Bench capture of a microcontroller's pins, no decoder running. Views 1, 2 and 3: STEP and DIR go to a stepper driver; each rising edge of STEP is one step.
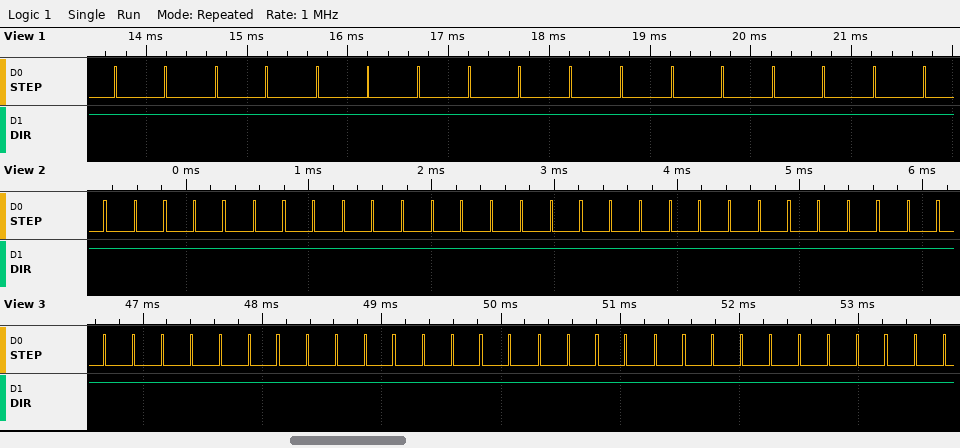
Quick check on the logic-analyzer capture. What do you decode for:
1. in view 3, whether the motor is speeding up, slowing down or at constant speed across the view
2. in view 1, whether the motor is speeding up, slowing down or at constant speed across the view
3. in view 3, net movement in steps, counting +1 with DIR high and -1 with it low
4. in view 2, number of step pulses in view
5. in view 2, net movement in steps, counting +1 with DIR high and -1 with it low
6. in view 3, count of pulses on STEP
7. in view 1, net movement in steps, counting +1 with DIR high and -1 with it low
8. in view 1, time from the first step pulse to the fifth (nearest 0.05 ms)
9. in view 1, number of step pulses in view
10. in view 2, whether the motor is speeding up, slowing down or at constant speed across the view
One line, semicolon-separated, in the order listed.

constant speed; constant speed; +30; 29; +29; 30; +17; 2.00 ms; 17; constant speed
